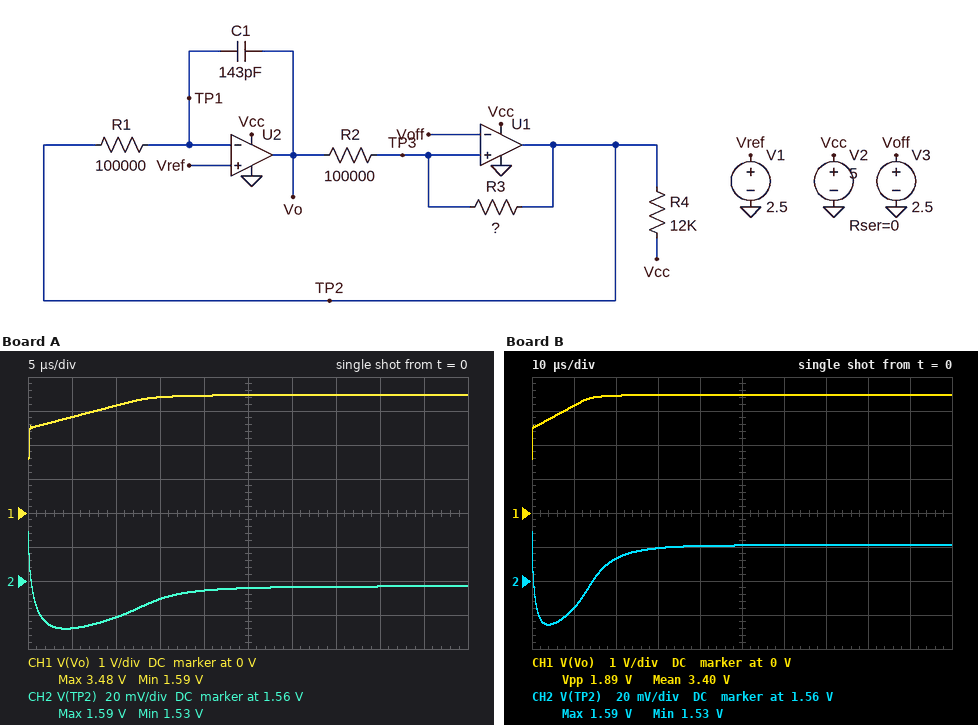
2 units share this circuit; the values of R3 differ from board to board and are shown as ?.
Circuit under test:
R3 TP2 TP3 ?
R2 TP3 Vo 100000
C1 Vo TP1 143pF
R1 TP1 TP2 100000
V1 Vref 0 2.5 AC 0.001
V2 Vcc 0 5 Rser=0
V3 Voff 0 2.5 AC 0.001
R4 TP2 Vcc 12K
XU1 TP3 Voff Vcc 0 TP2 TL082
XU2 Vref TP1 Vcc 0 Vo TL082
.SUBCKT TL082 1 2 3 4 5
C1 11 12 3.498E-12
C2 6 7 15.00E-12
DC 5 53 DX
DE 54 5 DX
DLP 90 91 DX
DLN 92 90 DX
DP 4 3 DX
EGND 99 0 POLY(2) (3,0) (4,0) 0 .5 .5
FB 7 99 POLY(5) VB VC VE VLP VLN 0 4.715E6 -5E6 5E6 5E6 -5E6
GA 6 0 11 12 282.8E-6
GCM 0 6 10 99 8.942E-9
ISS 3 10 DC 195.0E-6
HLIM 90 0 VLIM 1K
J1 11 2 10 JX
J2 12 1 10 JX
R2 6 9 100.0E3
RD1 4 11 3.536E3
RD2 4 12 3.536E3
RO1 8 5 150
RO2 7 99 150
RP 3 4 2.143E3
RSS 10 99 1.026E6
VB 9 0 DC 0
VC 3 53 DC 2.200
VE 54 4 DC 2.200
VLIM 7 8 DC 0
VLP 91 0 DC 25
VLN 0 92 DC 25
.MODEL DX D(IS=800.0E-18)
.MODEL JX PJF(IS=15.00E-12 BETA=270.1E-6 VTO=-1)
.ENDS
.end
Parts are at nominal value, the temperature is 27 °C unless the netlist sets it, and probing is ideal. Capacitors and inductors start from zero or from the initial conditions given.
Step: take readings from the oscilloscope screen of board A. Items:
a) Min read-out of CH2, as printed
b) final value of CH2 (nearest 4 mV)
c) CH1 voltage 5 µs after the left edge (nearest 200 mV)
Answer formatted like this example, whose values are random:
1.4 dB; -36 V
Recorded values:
1.53 V; 1.556 V; 2.8 V
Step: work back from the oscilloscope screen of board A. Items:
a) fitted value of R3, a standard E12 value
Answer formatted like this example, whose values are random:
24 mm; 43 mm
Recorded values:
68 kΩ
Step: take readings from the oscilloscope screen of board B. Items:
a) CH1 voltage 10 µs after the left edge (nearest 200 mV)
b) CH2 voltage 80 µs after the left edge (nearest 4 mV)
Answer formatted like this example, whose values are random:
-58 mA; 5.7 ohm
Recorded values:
3.2 V; 1.580 V
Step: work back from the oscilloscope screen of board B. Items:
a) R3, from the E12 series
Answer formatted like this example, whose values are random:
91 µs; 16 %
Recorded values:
82 kΩ
